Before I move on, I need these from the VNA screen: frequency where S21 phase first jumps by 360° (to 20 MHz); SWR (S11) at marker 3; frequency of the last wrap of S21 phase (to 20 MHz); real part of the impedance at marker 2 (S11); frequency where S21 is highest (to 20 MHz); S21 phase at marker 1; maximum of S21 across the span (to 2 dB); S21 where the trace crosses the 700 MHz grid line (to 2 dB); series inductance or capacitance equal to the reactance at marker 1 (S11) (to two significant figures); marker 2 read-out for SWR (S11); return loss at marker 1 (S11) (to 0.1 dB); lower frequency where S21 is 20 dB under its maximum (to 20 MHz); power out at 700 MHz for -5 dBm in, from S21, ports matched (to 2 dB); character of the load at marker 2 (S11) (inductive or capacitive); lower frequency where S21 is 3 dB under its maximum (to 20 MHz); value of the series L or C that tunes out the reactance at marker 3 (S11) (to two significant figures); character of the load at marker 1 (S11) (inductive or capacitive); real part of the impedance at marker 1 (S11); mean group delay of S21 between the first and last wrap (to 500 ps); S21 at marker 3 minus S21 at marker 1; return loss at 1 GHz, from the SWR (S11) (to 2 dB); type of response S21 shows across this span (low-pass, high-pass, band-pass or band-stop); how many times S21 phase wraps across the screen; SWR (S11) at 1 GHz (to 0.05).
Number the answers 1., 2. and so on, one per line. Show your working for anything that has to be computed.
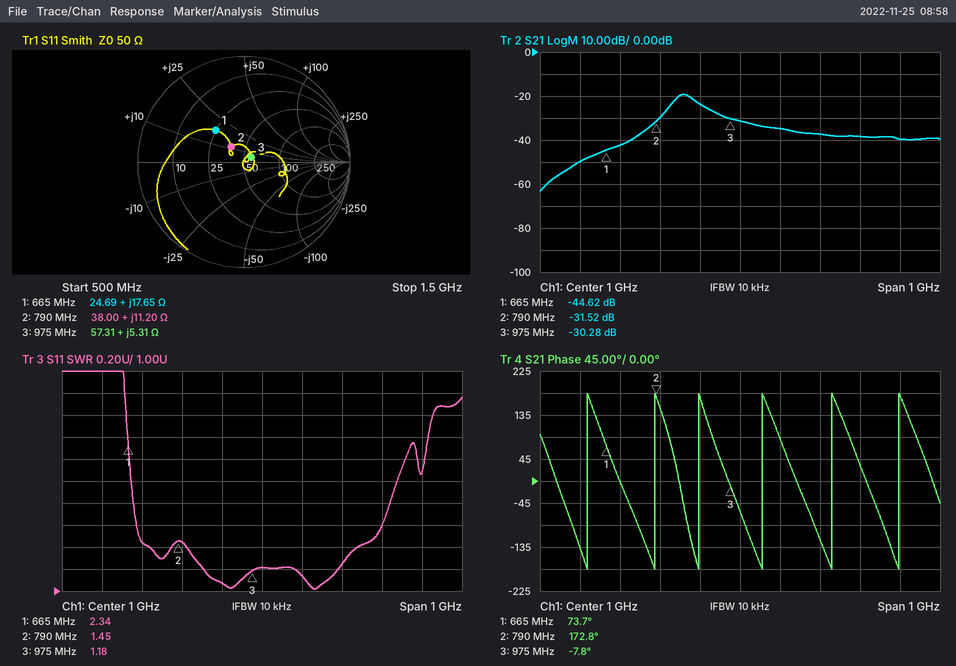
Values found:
1. 620 MHz
2. 1.18
3. 1.40 GHz
4. 38.00 Ω
5. 860 MHz
6. 73.7°
7. -20 dB
8. -42 dB
9. L = 17.65 Ω/(2π × 665 MHz) ≈ 4.2 nH
10. 1.45
11. 7.9 dB
12. 740 MHz
13. -5 dBm + (-42 dB) = -48 dBm
14. inductive
15. 840 MHz
16. C = 1/(2π × 975 MHz × 5.31 Ω) ≈ 31 pF
17. inductive
18. 24.69 Ω
19. 5 cycles / (1.40 GHz − 620 MHz) ≈ 6.41 ns, so 6.5 ns to the nearest 500 ps
20. -30.28 − (-44.62) = 14.34 dB
21. −20 log10((1.2 − 1)/(1.2 + 1)) ≈ 20.8 dB, so 20 dB to the nearest 2 dB
22. band-pass
23. 6
24. 1.20
